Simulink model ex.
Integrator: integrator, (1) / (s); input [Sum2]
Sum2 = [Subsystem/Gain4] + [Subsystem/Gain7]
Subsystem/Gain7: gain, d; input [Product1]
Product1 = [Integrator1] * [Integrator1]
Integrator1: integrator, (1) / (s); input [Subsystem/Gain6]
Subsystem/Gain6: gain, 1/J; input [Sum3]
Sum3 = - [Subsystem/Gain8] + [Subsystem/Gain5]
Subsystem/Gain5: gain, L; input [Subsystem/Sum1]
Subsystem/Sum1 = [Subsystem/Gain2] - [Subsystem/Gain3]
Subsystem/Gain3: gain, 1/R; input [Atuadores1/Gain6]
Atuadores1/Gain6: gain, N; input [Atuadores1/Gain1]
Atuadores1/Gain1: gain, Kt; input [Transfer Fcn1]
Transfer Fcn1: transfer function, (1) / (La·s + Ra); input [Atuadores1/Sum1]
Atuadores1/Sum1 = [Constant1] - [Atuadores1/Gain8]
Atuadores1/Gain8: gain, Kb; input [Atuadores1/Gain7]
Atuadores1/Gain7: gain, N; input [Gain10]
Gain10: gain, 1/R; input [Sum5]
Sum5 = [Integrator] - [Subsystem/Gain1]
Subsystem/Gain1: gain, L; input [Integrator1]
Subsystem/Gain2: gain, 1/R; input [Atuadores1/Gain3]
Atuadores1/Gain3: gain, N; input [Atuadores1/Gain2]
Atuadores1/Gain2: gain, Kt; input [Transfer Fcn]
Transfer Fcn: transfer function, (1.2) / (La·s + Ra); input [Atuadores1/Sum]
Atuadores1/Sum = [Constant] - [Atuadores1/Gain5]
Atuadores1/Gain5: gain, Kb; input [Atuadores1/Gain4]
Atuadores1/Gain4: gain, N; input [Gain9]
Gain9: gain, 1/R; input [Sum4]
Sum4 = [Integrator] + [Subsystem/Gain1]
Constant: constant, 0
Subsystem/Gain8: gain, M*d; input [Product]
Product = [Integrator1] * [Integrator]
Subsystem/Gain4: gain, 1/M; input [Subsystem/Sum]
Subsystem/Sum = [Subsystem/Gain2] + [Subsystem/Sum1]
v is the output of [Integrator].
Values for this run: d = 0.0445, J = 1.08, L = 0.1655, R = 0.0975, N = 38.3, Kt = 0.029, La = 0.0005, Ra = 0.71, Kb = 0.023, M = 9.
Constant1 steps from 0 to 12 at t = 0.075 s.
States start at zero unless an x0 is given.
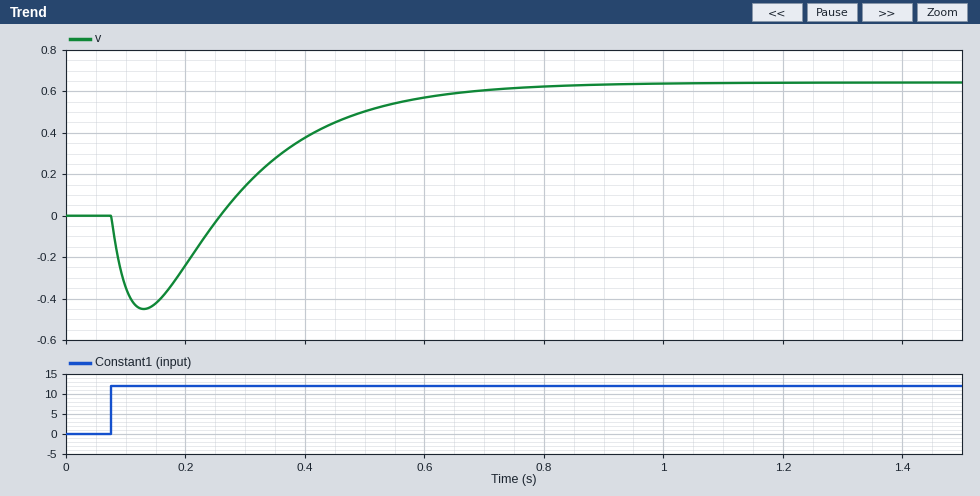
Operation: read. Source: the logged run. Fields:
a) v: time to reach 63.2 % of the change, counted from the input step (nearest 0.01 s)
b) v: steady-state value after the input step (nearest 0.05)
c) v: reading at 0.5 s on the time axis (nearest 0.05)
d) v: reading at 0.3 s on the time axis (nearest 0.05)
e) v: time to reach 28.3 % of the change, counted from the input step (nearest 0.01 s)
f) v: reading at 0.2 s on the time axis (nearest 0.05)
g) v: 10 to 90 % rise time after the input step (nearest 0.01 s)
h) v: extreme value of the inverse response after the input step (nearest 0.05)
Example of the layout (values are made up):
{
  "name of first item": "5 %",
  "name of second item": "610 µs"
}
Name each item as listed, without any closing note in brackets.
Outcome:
{
  "v: time to reach 63.2 % of the change, counted from the input step": "0.34 s",
  "v: steady-state value after the input step": "0.65",
  "v: reading at 0.5 s on the time axis": "0.50",
  "v: reading at 0.3 s on the time axis": "0.15",
  "v: time to reach 28.3 % of the change, counted from the input step": "0.24 s",
  "v: reading at 0.2 s on the time axis": "-0.25",
  "v: 10 to 90 % rise time after the input step": "0.34 s",
  "v: extreme value of the inverse response after the input step": "-0.45"
}
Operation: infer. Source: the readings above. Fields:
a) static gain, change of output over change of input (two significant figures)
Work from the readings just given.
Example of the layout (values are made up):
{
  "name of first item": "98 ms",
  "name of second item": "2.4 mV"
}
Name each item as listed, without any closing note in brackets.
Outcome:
{
  "static gain, change of output over change of input": "0.054"
}
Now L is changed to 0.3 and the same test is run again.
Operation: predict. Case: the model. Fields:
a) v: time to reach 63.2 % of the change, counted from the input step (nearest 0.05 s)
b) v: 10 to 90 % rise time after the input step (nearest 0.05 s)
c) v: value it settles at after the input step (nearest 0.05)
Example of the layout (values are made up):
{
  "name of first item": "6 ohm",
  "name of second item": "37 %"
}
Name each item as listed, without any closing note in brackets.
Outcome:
{
  "v: time to reach 63.2 % of the change, counted from the input step": "0.15 s",
  "v: 10 to 90 % rise time after the input step": "0.15 s",
  "v: value it settles at after the input step": "0.65"
}
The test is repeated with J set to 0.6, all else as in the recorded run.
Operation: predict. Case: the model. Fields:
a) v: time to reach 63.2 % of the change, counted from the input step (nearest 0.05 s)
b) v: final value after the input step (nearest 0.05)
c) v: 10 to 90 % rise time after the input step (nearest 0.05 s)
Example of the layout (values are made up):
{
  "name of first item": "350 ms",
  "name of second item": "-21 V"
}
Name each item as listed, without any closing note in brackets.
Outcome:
{
  "v: time to reach 63.2 % of the change, counted from the input step": "0.20 s",
  "v: final value after the input step": "0.65",
  "v: 10 to 90 % rise time after the input step": "0.20 s"
}
